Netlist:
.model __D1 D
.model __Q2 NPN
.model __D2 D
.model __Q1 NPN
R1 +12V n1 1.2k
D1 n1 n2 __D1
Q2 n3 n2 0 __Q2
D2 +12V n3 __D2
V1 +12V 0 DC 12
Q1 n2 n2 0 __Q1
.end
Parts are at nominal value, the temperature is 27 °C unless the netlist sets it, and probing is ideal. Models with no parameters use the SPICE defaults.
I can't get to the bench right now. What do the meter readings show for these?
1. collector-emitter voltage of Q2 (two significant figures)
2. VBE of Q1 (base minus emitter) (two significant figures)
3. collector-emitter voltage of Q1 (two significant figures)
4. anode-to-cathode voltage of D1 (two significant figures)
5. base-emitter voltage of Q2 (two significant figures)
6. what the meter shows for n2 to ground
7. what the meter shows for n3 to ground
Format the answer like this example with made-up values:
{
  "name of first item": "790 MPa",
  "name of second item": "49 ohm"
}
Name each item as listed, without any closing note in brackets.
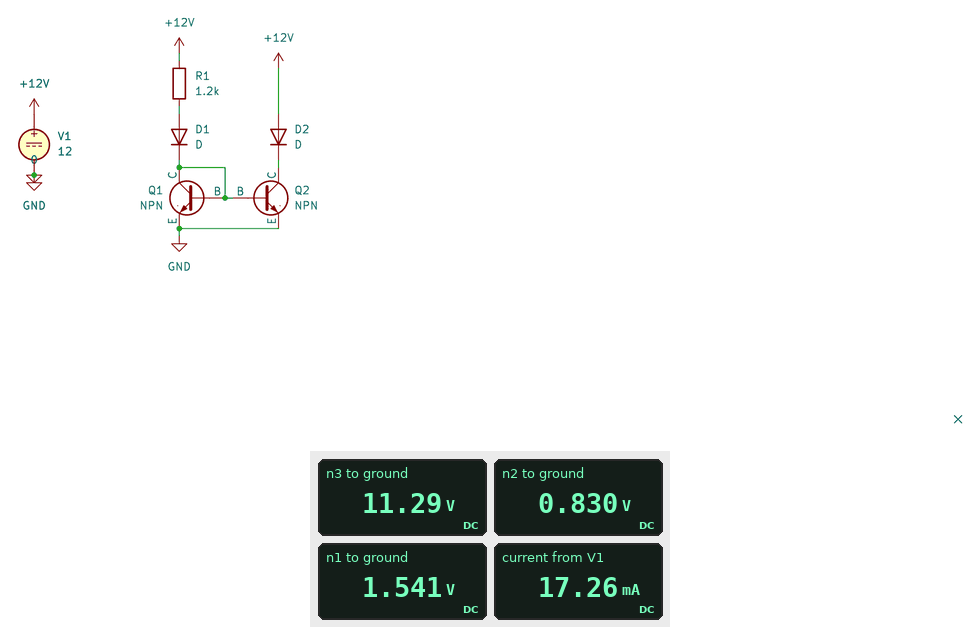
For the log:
{
  "collector-emitter voltage of Q2": "11 V",
  "VBE of Q1 (base minus emitter)": "830 mV",
  "collector-emitter voltage of Q1": "830 mV",
  "anode-to-cathode voltage of D1": "710 mV",
  "base-emitter voltage of Q2": "830 mV",
  "what the meter shows for n2 to ground": "0.830 V",
  "what the meter shows for n3 to ground": "11.29 V"
}
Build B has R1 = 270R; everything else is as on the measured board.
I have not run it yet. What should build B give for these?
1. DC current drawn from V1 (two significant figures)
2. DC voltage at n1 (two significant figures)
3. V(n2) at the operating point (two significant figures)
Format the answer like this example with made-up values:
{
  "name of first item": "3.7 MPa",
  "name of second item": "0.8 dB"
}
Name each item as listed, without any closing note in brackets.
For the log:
{
  "DC current drawn from V1": "76 mA",
  "DC voltage at n1": "1.6 V",
  "V(n2) at the operating point": "870 mV"
}
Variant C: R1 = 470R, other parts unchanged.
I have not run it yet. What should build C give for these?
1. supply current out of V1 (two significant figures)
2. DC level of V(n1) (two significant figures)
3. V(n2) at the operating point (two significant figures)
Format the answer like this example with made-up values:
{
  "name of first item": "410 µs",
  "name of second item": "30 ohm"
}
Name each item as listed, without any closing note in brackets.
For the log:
{
  "supply current out of V1": "44 mA",
  "DC level of V(n1)": "1.6 V",
  "V(n2) at the operating point": "850 mV"
}
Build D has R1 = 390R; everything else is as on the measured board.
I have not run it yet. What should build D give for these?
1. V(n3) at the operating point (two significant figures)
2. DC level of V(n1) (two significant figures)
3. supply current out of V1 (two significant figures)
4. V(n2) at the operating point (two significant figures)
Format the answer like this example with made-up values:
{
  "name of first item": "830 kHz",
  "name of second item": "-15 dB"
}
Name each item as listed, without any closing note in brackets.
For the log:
{
  "V(n3) at the operating point": "11 V",
  "DC level of V(n1)": "1.6 V",
  "supply current out of V1": "53 mA",
  "V(n2) at the operating point": "860 mV"
}
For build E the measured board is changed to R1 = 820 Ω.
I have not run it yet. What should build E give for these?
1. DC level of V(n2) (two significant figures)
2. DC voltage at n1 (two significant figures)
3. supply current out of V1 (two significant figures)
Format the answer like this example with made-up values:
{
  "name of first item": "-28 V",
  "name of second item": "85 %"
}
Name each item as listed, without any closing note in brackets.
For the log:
{
  "DC level of V(n2)": "840 mV",
  "DC voltage at n1": "1.6 V",
  "supply current out of V1": "25 mA"
}
